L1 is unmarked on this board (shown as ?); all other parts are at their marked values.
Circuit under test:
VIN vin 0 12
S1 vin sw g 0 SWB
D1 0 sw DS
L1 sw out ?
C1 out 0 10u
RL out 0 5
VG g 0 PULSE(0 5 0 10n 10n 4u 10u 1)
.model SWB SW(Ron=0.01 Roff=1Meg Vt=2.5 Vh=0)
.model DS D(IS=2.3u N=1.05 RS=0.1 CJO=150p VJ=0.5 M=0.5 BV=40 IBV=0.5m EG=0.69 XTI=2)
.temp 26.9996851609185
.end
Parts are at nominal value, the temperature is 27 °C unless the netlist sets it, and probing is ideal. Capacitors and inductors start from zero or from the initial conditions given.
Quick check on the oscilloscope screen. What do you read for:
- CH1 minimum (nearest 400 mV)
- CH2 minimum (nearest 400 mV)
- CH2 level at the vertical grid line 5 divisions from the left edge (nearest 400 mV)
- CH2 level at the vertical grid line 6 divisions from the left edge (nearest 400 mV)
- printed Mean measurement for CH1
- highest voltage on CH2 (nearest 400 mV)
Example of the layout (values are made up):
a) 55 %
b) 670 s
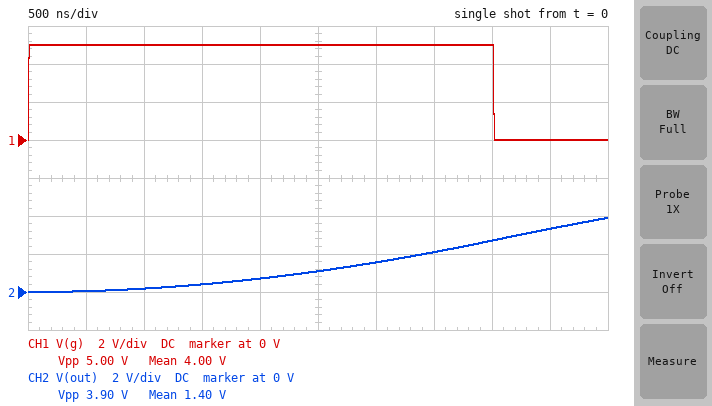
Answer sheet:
a) 0 V
b) 0 V
c) 1.2 V
d) 1.6 V
e) 4.00 V
f) 4.0 V
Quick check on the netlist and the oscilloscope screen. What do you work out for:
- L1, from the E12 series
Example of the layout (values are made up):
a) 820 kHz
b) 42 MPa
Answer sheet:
a) 3.3 µH
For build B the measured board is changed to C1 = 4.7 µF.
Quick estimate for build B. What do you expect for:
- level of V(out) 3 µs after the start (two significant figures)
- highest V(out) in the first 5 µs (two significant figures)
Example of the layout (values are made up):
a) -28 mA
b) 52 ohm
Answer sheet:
a) 3.2 V
b) 7.4 V
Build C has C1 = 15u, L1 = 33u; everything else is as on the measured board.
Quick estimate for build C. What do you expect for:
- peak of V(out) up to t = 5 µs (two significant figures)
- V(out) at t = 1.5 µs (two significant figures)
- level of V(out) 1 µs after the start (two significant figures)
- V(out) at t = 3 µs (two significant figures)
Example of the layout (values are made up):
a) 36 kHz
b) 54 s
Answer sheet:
a) 280 mV
b) 27 mV
c) 12 mV
d) 110 mV
